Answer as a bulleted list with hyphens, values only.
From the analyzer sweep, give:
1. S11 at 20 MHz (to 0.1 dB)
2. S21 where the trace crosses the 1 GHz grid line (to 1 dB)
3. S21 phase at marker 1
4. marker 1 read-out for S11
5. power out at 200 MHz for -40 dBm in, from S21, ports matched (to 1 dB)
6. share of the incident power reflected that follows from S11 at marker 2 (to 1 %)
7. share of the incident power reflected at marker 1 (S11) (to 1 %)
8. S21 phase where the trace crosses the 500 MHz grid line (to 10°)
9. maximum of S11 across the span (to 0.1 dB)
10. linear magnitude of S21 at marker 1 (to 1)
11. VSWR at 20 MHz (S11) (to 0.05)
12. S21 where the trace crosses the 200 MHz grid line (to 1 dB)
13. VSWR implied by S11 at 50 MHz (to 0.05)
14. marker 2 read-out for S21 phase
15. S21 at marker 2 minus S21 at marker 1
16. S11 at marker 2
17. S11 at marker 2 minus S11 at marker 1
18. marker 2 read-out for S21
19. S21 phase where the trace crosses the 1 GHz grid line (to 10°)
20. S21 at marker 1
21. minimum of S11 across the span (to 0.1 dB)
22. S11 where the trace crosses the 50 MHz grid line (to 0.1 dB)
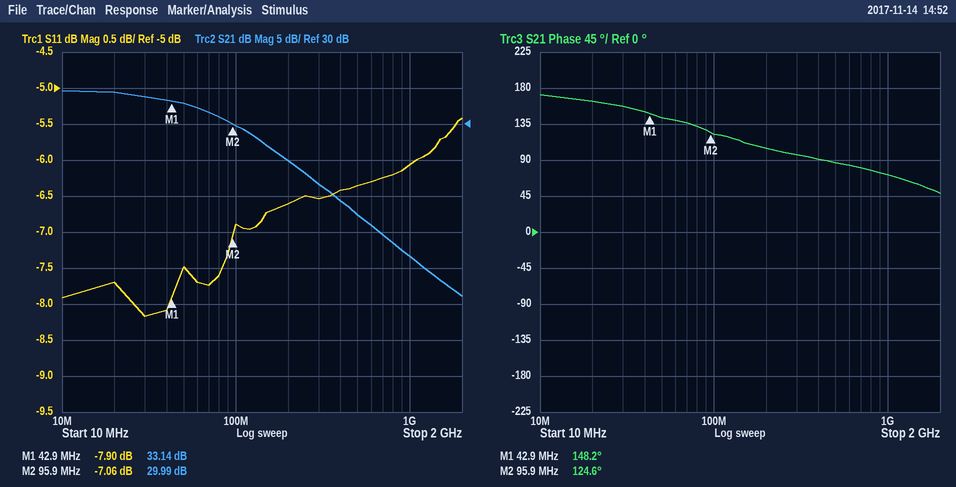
- -7.7 dB
- 12 dB
- 148.2°
- -7.90 dB
- -15 dBm
- 20 %
- 16 %
- 90°
- -5.4 dB
- 45
- 2.40
- 25 dB
- 2.45
- 124.6°
- -3.15 dB
- -7.06 dB
- 0.84 dB
- 29.99 dB
- 70°
- 33.14 dB
- -8.2 dB
- -7.5 dB
